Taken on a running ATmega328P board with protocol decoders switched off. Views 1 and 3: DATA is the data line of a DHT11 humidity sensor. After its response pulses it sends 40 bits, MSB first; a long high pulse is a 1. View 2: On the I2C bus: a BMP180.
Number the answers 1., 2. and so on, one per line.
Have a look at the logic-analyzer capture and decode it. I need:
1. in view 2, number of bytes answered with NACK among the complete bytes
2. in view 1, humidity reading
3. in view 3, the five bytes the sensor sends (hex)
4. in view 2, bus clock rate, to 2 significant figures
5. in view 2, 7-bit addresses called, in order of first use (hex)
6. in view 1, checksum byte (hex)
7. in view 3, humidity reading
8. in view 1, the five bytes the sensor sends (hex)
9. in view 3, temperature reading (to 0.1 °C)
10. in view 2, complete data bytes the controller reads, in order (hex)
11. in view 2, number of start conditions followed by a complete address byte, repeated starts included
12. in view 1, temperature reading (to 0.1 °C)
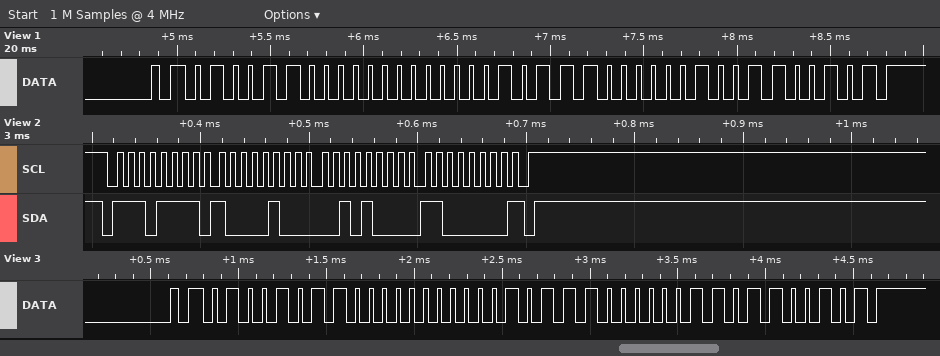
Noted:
1. 1
2. 76 %
3. 4B 00 17 03 65
4. 100 kHz
5. 0x77
6. 0x65
7. 75 %
8. 4C 00 17 02 65
9. 23.3 °C
10. 84 28 C0
11. 1
12. 23.2 °C
